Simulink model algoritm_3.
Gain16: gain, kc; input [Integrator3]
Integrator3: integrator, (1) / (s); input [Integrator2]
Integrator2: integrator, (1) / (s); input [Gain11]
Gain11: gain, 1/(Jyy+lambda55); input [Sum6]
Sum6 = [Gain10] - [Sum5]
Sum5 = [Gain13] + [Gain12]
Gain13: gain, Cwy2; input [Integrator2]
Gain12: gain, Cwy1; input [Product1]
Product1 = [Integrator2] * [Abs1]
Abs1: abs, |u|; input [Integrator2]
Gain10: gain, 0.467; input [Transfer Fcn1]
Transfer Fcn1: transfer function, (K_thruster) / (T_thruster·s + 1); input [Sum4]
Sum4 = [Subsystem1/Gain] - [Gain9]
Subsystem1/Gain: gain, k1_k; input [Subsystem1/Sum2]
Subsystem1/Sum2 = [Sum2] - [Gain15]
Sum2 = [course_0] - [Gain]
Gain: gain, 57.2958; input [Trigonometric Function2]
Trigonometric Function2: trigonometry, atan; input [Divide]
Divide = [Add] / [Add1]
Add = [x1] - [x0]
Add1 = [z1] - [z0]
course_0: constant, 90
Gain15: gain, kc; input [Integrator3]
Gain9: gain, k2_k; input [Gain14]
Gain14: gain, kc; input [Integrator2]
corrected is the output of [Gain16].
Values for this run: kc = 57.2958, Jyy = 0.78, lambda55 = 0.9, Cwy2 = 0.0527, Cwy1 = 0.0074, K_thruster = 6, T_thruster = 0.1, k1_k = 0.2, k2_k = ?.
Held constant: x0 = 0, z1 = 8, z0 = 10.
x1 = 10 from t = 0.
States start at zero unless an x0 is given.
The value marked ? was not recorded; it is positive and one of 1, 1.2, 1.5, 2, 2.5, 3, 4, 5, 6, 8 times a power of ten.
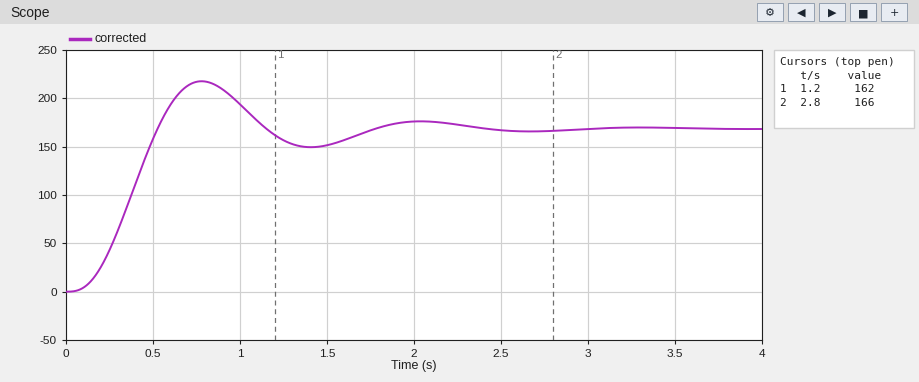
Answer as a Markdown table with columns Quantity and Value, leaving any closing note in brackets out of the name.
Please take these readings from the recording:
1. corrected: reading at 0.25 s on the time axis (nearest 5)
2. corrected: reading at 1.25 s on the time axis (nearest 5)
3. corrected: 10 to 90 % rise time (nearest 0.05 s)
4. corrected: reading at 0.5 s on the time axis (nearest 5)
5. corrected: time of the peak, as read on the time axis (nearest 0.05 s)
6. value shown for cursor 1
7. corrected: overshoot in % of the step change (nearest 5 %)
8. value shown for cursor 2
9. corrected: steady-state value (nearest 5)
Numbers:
| Quantity | Value |
|---|---|
| corrected: reading at 0.25 s on the time axis | 45 |
| corrected: reading at 1.25 s on the time axis | 155 |
| corrected: 10 to 90 % rise time | 0.30 s |
| corrected: reading at 0.5 s on the time axis | 160 |
| corrected: time of the peak, as read on the time axis | 0.80 s |
| value shown for cursor 1 | 162 |
| corrected: overshoot in % of the step change | 30 % |
| value shown for cursor 2 | 166 |
| corrected: steady-state value | 170 |
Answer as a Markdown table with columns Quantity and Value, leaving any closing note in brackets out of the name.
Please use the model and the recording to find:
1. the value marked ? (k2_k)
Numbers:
| Quantity | Value |
|---|---|
| the value marked ? | 0.05 |
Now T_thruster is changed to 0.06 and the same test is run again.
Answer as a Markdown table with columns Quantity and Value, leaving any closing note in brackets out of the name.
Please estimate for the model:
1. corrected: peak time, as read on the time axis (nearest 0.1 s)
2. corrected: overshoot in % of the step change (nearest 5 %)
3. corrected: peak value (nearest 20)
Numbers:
| Quantity | Value |
|---|---|
| corrected: peak time, as read on the time axis | 0.8 s |
| corrected: overshoot in % of the step change | 20 % |
| corrected: peak value | 200 |
